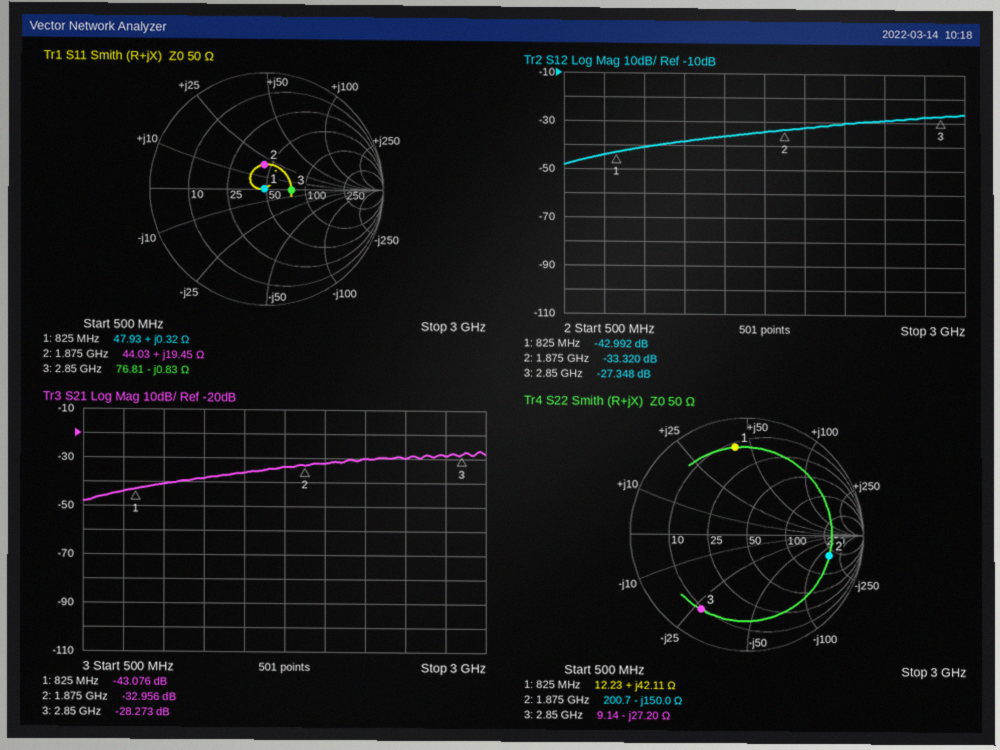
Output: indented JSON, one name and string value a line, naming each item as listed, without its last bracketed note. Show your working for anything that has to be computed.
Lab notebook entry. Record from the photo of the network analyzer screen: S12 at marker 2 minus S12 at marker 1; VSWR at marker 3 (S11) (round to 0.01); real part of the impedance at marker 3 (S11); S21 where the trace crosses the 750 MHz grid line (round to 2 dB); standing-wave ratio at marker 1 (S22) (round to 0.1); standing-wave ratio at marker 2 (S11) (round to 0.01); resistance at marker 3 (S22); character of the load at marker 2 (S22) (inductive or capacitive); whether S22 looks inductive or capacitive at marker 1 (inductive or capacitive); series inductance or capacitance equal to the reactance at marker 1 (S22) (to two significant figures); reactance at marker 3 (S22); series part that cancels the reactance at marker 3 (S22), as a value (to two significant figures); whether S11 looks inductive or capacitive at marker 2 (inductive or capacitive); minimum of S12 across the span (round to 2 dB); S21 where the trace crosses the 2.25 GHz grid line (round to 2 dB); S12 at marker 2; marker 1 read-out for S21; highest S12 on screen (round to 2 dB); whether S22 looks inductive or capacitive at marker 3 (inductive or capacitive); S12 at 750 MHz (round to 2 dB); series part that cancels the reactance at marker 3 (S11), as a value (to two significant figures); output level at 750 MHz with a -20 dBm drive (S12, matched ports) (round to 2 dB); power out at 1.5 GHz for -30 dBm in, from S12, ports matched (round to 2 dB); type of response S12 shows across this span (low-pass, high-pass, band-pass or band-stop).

{
  "S12 at marker 2 minus S12 at marker 1": "-33.32 − (-42.992) = 9.672 dB",
  "VSWR at marker 3 (S11)": "1.54",
  "real part of the impedance at marker 3": "76.81 Ω",
  "S21 where the trace crosses the 750 MHz grid line": "-44 dB",
  "standing-wave ratio at marker 1 (S22)": "7.1",
  "standing-wave ratio at marker 2 (S11)": "1.54",
  "resistance at marker 3": "9.14 Ω",
  "character of the load at marker 2 (S22)": "capacitive",
  "whether S22 looks inductive or capacitive at marker 1": "inductive",
  "series inductance or capacitance equal to the reactance at marker 1 (S22)": "L = 42.11 Ω/(2π × 825 MHz) ≈ 8.1 nH",
  "reactance at marker 3": "-27.20 Ω",
  "series part that cancels the reactance at marker 3 (S22), as a value": "L = 27.2 Ω/(2π × 2.85 GHz) ≈ 1.5 nH",
  "whether S11 looks inductive or capacitive at marker 2": "inductive",
  "minimum of S12 across the span": "-48 dB",
  "S21 where the trace crosses the 2.25 GHz grid line": "-30 dB",
  "S12 at marker 2": "-33.320 dB",
  "marker 1 read-out for S21": "-43.076 dB",
  "highest S12 on screen": "-26 dB",
  "whether S22 looks inductive or capacitive at marker 3": "capacitive",
  "S12 at 750 MHz": "-44 dB",
  "series part that cancels the reactance at marker 3 (S11), as a value": "L = 0.83 Ω/(2π × 2.85 GHz) ≈ 46 pH",
  "output level at 750 MHz with a -20 dBm drive (S12, matched ports)": "-20 dBm + (-44 dB) = -64 dBm",
  "power out at 1.5 GHz for -30 dBm in, from S12, ports matched": "-30 dBm + (-36 dB) = -66 dBm",
  "type of response S12 shows across this span": "high-pass"
}
